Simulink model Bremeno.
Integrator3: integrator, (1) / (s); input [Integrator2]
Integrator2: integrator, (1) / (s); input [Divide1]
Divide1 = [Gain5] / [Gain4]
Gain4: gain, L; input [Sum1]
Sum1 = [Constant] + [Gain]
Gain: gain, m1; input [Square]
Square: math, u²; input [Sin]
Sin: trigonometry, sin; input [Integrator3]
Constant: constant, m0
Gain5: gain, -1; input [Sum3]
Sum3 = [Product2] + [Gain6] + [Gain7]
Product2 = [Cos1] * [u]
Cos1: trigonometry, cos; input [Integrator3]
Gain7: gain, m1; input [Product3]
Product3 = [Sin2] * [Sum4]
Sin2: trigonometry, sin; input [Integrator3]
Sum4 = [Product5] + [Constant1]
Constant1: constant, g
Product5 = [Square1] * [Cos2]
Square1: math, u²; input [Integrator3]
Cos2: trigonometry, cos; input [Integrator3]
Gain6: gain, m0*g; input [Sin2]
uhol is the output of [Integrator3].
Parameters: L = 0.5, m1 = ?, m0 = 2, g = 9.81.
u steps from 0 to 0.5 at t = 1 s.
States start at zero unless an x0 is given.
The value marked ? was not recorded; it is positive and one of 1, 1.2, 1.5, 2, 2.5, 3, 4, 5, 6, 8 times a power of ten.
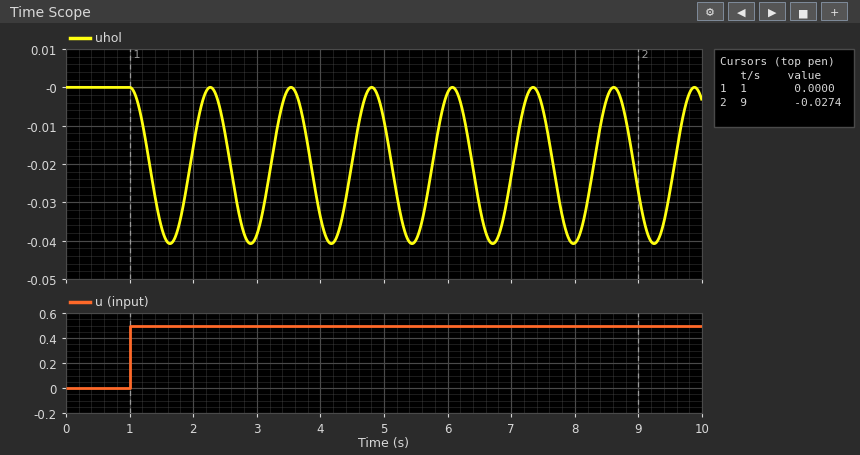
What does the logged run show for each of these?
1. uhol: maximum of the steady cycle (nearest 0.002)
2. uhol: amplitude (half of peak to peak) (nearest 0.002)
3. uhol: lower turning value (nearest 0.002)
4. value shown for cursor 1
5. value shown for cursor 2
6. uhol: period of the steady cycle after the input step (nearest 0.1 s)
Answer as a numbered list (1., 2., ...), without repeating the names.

1. 0.000
2. 0.020
3. -0.040
4. 0.0000
5. -0.0274
6. 1.3 s
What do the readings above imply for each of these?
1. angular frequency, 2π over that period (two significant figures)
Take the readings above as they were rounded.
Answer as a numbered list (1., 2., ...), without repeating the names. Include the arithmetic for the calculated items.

1. 2π / 1.3 = 4.8 rad/s
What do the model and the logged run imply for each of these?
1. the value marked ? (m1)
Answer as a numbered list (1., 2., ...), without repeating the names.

1. 0.5
